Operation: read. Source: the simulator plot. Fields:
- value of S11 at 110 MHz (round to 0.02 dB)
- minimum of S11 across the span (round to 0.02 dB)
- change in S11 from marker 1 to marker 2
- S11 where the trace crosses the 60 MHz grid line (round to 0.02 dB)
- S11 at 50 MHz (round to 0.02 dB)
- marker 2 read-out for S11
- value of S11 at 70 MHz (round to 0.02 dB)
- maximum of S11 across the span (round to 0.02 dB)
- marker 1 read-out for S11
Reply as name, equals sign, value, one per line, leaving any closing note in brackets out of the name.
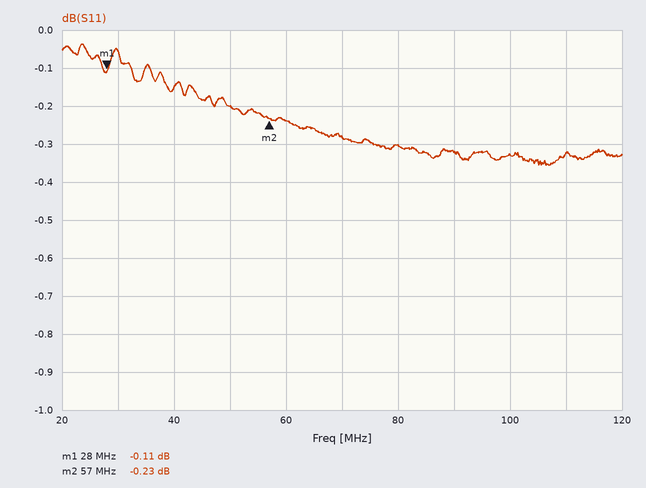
value of S11 at 110 MHz = -0.32 dB
minimum of S11 across the span = -0.36 dB
change in S11 from marker 1 to marker 2 = -0.12 dB
S11 where the trace crosses the 60 MHz grid line = -0.24 dB
S11 at 50 MHz = -0.20 dB
marker 2 read-out for S11 = -0.23 dB
value of S11 at 70 MHz = -0.28 dB
maximum of S11 across the span = -0.04 dB
marker 1 read-out for S11 = -0.11 dB
